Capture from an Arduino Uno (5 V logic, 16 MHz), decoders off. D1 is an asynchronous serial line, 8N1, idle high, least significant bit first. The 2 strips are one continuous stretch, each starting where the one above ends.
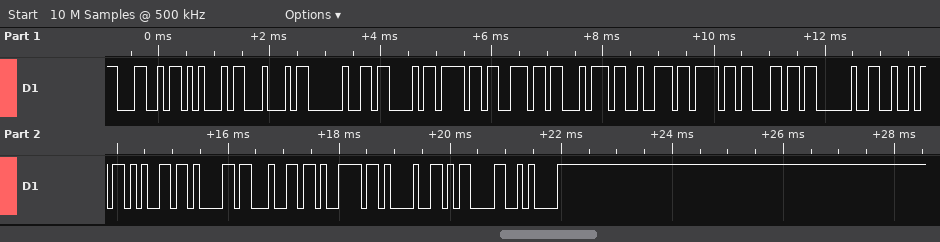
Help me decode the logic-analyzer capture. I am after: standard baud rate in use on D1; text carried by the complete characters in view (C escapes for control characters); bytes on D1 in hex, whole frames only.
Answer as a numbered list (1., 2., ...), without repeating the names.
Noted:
1. 9600 baud
2. "LED Control Ready!\r\n"
3. 0x4C 0x45 0x44 0x20 0x43 0x6F 0x6E 0x74 0x72 0x6F 0x6C 0x20 0x52 0x65 0x61 0x64 0x79 0x21 0x0D 0x0A
